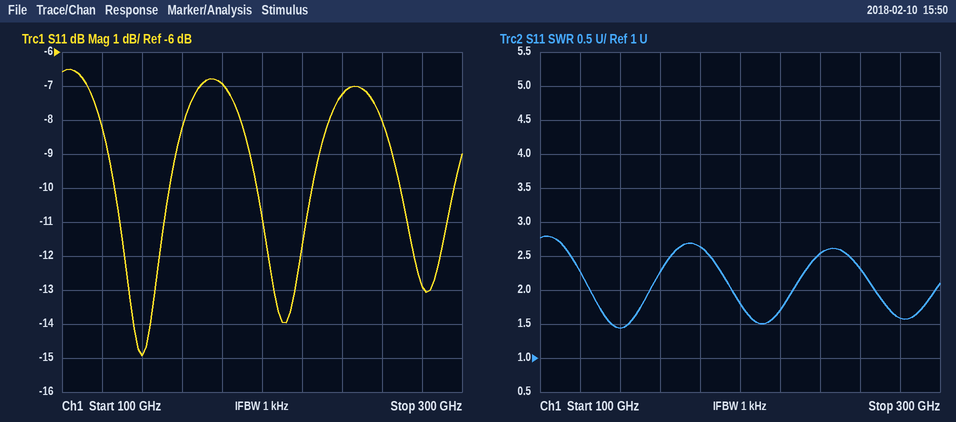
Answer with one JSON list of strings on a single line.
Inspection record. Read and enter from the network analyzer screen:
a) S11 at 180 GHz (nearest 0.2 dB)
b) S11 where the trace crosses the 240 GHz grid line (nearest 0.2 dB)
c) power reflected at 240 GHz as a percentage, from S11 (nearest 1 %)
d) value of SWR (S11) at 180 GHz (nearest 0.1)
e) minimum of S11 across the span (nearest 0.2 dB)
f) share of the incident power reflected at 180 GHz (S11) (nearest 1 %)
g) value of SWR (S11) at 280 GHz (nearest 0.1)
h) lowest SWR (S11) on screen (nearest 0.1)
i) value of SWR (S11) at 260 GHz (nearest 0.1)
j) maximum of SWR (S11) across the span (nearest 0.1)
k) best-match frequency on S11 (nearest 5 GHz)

["-7.0 dB", "-7.2 dB", "19 %", "2.6", "-15.0 dB", "20 %", "1.6", "1.4", "2.3", "2.8", "140 GHz"]
